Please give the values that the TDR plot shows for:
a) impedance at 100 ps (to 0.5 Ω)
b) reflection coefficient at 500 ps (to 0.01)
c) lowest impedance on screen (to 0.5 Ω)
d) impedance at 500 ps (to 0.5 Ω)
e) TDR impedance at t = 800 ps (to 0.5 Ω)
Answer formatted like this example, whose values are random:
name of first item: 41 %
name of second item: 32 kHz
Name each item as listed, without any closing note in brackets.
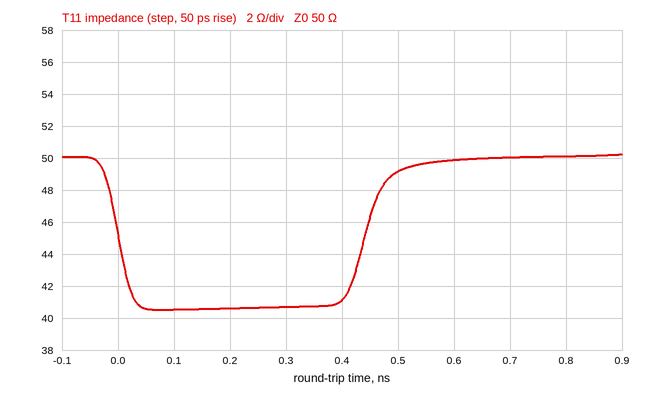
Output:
impedance at 100 ps: 40.5 Ω
reflection coefficient at 500 ps: -0.01
lowest impedance on screen: 40.5 Ω
impedance at 500 ps: 49.0 Ω
TDR impedance at t = 800 ps: 50.0 Ω
